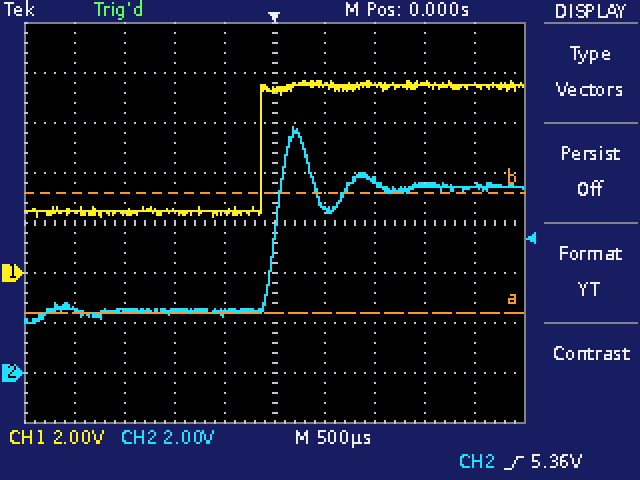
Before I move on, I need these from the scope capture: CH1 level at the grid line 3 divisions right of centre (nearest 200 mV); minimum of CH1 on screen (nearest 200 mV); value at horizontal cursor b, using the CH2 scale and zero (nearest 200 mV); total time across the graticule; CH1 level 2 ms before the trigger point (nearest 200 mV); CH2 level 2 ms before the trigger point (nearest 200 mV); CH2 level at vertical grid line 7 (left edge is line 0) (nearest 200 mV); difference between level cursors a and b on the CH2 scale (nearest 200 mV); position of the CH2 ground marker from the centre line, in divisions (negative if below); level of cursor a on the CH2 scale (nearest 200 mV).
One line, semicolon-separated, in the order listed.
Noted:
7.6 V; 2.2 V; 7.2 V; 5 ms; 2.4 V; 2.6 V; 7.6 V; 4.8 V; -3.0 div; 2.4 V
